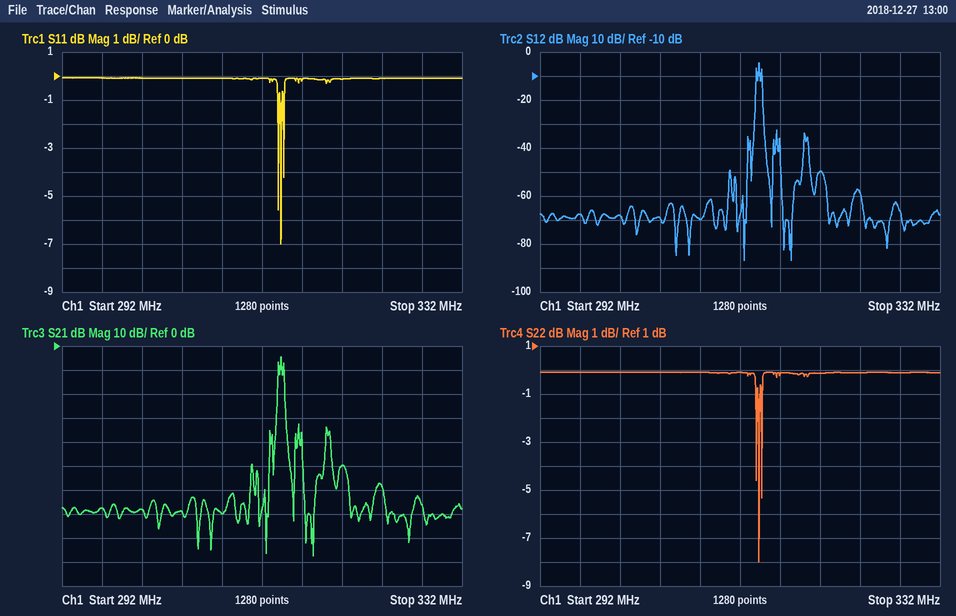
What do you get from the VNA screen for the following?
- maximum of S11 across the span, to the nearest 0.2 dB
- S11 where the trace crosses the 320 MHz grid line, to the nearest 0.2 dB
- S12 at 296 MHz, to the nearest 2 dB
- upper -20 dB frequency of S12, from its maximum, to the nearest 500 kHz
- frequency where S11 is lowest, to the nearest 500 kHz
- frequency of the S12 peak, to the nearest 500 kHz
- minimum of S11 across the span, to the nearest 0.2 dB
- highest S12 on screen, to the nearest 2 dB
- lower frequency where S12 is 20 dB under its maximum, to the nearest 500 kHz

0.0 dB
-0.2 dB
-68 dB
314.5 MHz
314.0 MHz
314.0 MHz
-7.0 dB
-4 dB
313.5 MHz
